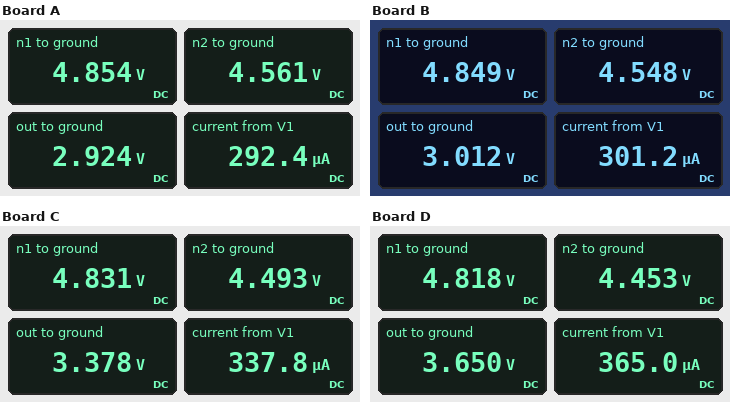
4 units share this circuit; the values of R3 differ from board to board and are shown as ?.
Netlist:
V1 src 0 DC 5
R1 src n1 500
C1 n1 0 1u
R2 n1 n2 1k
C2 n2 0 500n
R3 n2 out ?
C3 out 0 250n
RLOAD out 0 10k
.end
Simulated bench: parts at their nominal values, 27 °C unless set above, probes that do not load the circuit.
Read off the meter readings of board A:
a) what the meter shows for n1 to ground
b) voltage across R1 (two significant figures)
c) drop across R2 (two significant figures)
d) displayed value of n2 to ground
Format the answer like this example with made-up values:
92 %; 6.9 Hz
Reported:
4.854 V; 150 mV; 290 mV; 4.561 V
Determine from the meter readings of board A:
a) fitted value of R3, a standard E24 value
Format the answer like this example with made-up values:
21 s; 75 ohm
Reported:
5.6 kΩ
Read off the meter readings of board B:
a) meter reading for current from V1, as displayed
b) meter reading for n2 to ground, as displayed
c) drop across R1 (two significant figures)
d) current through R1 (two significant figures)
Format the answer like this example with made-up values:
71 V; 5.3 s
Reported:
301.2 µA; 4.548 V; 150 mV; 300 µA
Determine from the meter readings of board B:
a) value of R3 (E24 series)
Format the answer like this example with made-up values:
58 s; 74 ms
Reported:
5.1 kΩ
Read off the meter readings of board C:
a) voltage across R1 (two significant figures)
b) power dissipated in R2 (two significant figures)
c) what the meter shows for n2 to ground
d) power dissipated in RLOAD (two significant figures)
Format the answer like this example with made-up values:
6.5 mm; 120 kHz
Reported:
170 mV; 110 µW; 4.493 V; 1.1 mW
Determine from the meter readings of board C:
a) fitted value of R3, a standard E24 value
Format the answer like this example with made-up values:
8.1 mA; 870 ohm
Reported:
3.3 kΩ
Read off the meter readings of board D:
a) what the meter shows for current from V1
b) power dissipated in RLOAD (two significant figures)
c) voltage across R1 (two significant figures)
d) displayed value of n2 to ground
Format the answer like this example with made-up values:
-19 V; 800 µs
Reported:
365.0 µA; 1.3 mW; 180 mV; 4.453 V
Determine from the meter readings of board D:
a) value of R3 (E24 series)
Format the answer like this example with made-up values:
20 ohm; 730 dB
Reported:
2.2 kΩ
